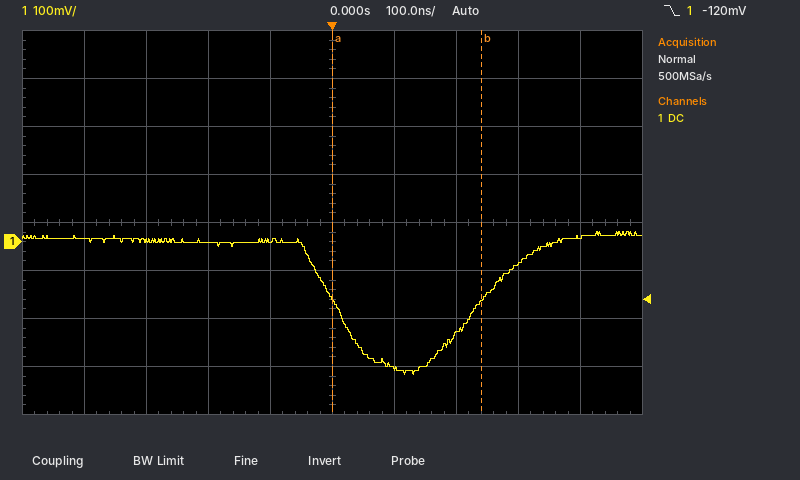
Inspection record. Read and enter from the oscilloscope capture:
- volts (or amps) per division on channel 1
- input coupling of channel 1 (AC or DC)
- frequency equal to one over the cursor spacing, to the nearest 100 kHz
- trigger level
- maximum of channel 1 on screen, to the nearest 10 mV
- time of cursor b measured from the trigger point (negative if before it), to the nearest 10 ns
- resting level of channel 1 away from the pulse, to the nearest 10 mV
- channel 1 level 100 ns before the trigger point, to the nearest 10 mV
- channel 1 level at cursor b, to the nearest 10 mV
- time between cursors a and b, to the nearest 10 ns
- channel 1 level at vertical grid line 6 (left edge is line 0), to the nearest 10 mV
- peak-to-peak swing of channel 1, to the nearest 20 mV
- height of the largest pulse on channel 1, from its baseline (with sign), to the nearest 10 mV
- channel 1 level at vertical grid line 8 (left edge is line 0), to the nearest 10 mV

100 mV
DC
4.2 MHz
-120 mV
20 mV
+240 ns
0 mV
0 mV
-120 mV
240 ns
-260 mV
300 mV
-280 mV
-50 mV
